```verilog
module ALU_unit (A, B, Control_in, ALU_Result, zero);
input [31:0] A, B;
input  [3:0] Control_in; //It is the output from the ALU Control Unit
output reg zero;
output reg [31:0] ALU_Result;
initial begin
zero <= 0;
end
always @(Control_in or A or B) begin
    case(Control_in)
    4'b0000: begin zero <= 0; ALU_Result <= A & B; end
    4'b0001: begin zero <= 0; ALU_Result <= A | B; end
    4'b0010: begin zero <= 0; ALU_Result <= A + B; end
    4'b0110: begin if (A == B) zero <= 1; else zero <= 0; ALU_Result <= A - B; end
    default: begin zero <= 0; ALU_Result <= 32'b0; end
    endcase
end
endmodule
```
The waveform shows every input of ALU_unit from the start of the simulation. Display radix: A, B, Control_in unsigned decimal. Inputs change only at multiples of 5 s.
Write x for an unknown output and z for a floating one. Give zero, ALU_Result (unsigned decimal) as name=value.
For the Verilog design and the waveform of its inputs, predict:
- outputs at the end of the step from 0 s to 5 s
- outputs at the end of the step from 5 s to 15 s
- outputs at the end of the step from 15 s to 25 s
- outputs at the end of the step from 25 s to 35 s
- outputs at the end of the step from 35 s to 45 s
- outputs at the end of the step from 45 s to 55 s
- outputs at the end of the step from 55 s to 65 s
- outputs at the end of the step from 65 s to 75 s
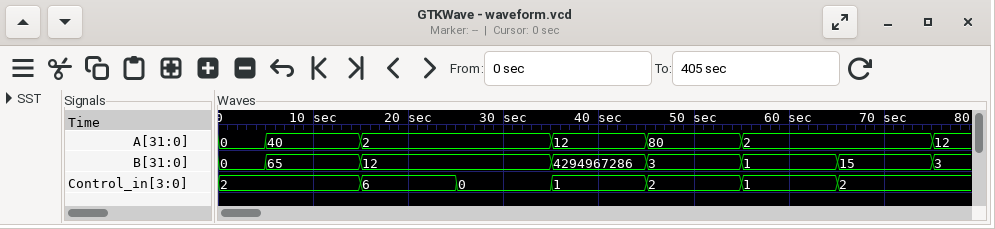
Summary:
zero=0, ALU_Result=0
zero=0, ALU_Result=105
zero=0, ALU_Result=4294967286
zero=0, ALU_Result=0
zero=0, ALU_Result=4294967294
zero=0, ALU_Result=83
zero=0, ALU_Result=3
zero=0, ALU_Result=17
